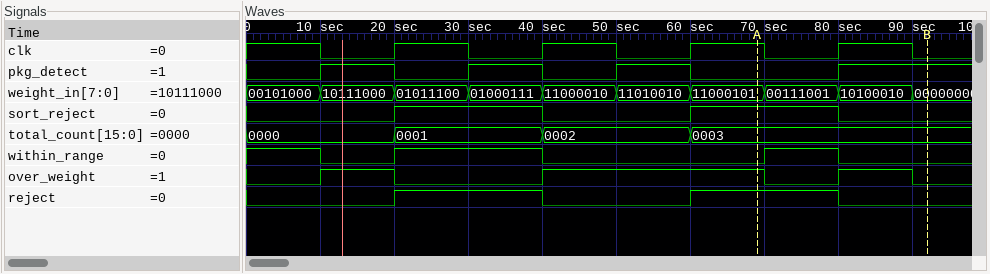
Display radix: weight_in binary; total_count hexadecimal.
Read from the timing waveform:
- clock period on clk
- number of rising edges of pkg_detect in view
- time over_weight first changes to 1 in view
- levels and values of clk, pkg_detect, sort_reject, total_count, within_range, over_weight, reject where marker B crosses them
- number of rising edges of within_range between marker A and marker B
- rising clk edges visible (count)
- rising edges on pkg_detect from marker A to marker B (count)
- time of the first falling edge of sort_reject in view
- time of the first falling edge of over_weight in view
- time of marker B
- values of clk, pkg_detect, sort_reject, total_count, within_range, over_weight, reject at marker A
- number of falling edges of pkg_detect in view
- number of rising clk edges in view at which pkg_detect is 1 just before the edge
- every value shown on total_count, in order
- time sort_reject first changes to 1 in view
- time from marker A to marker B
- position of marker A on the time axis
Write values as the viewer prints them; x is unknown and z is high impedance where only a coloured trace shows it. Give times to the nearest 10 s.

20 s
4
10 s
clk=0, pkg_detect=1, sort_reject=0, total_count=0003, within_range=0, over_weight=0, reject=0
1
4
1
40 s
20 s
90 s
clk=1, pkg_detect=0, sort_reject=1, total_count=0003, within_range=0, over_weight=1, reject=1
3
3
0000, 0001, 0002, 0003
20 s
20 s
70 s
